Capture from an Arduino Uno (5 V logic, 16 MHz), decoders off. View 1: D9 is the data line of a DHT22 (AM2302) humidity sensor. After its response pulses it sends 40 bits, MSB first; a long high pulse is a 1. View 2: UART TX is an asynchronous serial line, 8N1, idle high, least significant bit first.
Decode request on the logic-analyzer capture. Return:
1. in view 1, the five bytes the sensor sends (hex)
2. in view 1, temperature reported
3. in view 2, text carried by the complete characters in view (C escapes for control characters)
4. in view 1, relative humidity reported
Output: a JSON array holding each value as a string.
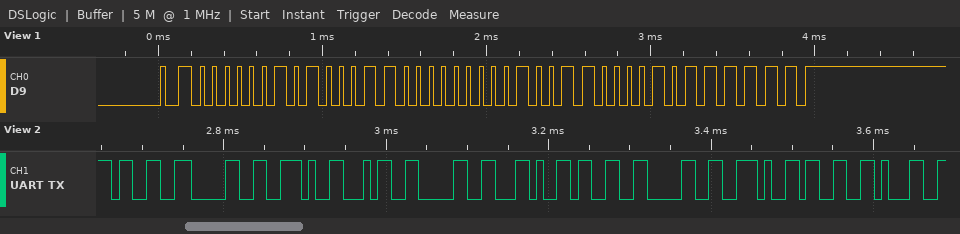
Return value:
["02 8C 01 30 BF", "30.4 °C", "\"30.40,30.31\"", "65.2 %"]
